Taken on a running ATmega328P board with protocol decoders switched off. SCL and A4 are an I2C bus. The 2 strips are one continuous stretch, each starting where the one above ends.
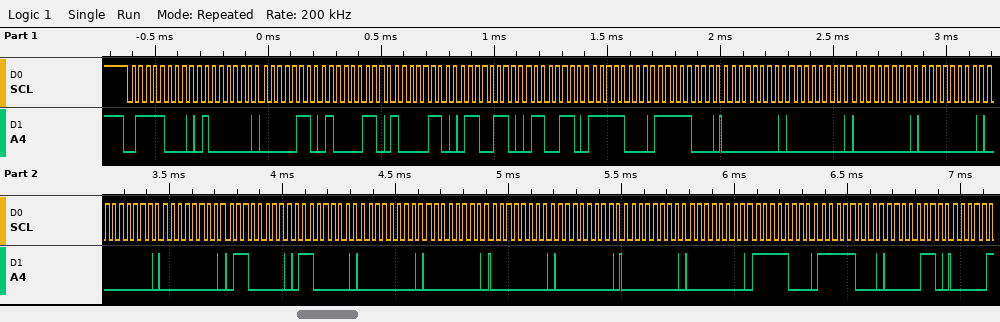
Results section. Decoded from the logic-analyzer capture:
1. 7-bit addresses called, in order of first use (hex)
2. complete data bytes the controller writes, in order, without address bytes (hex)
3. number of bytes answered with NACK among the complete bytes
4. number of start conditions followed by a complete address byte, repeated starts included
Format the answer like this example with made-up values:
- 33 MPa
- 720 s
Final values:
- 0x3C
- 40 06 86 86 66 66 F8 F8 00 00 00 00 00 00 60 60 00 00 00 00 00 00 F8 F8 06
- 0
- 1
